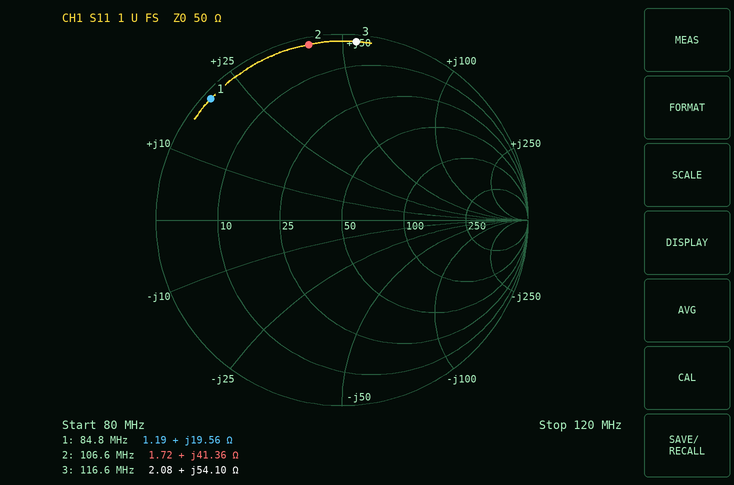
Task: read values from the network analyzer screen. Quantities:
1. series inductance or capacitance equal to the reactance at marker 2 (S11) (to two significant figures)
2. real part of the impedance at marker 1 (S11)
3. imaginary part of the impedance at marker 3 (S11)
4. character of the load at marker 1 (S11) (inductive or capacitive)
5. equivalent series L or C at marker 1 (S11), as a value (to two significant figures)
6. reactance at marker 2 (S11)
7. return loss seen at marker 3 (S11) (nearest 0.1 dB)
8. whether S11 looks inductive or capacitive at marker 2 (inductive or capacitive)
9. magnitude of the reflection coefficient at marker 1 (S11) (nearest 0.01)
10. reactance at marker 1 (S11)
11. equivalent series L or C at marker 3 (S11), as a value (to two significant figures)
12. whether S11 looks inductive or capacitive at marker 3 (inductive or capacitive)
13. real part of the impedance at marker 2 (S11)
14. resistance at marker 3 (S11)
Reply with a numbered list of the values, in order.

1. 62 nH
2. 1.19 Ω
3. +54.10 Ω
4. inductive
5. 37 nH
6. +41.36 Ω
7. 0.3 dB
8. inductive
9. 0.96
10. +19.56 Ω
11. 74 nH
12. inductive
13. 1.72 Ω
14. 2.08 Ω
